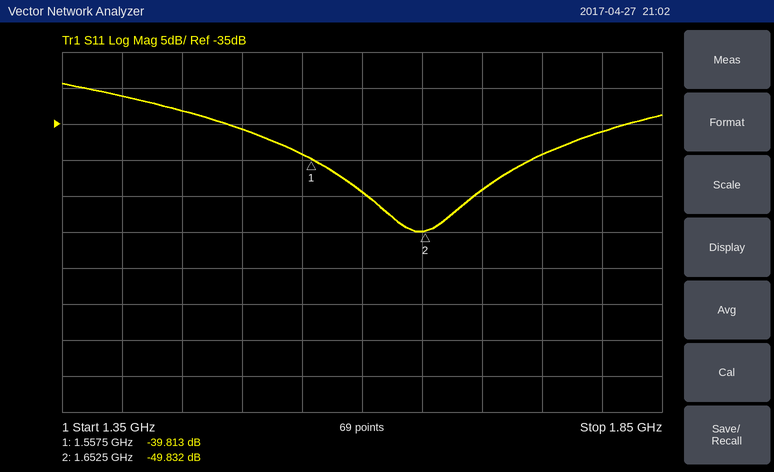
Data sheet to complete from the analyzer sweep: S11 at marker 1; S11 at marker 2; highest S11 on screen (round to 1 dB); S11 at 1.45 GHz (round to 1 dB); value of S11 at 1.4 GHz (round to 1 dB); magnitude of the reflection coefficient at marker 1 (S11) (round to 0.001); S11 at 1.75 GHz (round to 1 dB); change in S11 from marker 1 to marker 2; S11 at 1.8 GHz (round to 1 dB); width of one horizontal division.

-39.813 dB
-49.832 dB
-29 dB
-33 dB
-31 dB
0.010
-39 dB
-10.019 dB
-36 dB
50 MHz
